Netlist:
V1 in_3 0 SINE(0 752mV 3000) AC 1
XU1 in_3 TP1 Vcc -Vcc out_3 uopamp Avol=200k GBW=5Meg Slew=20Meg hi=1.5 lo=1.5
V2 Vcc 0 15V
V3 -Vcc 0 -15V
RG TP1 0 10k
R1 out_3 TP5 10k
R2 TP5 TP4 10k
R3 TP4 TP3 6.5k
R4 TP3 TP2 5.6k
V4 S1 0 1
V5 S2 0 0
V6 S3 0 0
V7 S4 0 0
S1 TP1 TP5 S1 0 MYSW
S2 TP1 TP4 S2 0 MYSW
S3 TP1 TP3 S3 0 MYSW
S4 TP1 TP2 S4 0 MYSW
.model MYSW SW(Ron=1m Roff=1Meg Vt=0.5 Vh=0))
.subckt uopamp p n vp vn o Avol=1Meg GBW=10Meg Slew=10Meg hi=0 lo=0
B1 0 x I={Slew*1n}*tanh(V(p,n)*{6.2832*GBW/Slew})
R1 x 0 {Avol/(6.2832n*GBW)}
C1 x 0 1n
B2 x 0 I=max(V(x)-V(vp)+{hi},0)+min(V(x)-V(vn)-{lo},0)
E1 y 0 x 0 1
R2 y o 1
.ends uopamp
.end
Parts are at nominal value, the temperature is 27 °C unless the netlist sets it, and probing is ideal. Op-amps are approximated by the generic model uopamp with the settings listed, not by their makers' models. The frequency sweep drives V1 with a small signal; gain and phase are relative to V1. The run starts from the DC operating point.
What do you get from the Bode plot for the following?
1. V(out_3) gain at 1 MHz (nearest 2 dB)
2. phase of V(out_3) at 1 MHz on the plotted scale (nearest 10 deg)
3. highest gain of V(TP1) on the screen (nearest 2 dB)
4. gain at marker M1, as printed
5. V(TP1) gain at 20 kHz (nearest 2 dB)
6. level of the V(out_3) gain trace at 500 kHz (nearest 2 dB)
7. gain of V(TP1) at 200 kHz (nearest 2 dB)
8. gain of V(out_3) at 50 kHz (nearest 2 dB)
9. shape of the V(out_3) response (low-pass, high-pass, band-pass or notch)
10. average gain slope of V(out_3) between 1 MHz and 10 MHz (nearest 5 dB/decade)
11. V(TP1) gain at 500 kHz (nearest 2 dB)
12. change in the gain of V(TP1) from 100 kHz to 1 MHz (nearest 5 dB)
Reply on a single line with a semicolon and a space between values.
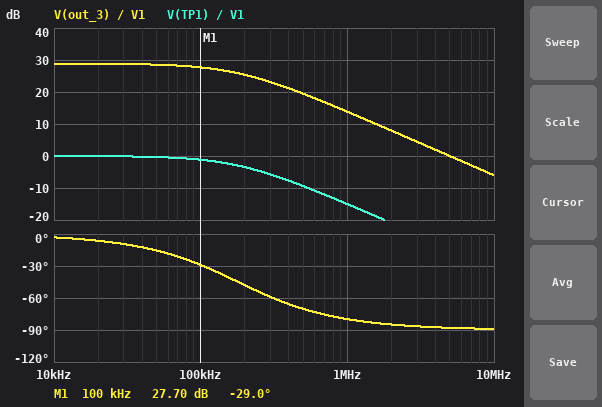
14 dB; -80 deg; 0 dB; 27.70 dB; 0 dB; 20 dB; -4 dB; 28 dB; low-pass; -20 dB/decade; -10 dB; -15 dB
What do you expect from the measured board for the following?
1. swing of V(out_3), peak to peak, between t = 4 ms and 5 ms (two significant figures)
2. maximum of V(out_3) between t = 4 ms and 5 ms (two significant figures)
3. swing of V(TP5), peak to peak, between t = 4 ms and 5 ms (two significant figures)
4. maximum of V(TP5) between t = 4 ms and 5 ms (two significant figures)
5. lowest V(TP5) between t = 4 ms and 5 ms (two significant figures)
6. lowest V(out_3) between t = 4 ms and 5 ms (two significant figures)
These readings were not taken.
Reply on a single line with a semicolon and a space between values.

3.0 V; 1.5 V; 1.5 V; 750 mV; -750 mV; -1.5 V
